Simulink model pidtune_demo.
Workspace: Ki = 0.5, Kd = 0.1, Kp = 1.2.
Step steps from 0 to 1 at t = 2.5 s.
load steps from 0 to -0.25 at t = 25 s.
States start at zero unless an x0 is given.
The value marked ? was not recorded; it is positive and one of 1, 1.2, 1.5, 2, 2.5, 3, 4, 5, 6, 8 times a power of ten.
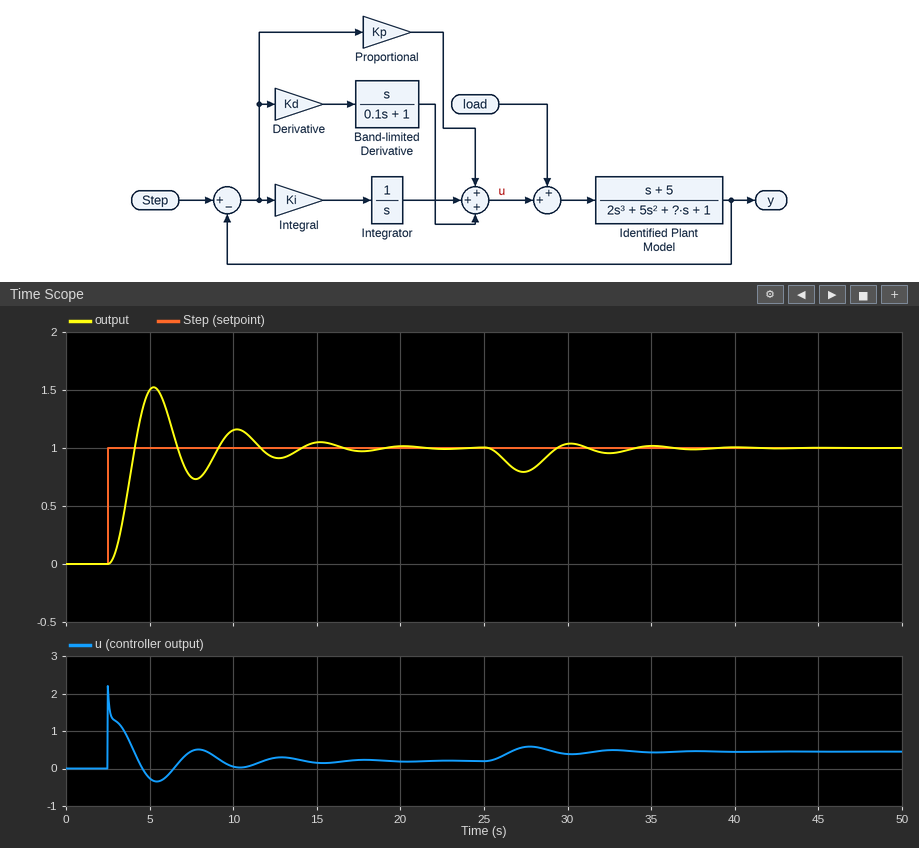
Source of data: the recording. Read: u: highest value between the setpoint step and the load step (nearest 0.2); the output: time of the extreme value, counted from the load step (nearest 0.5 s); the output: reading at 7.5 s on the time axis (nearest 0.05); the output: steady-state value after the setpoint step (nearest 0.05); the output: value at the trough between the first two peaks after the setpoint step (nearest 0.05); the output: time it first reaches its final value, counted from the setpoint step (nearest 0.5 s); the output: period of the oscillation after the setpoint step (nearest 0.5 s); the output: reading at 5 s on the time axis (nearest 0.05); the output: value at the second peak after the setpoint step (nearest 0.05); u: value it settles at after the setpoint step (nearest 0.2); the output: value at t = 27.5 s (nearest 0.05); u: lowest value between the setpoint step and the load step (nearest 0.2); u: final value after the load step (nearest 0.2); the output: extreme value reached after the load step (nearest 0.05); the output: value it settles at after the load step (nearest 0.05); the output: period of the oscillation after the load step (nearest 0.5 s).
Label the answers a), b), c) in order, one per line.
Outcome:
a) 2.2
b) 2.5 s
c) 0.75
d) 1.00
e) 0.75
f) 1.5 s
g) 5.0 s
h) 1.50
i) 1.15
j) 0.2
k) 0.80
l) -0.4
m) 0.4
n) 0.80
o) 1.00
p) 5.0 s
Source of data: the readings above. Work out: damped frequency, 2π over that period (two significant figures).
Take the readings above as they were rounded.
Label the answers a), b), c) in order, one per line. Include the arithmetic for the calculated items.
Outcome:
a) 2π / 5 = 1.3 rad/s
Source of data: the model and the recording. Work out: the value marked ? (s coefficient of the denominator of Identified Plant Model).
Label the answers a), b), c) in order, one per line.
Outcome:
a) 5
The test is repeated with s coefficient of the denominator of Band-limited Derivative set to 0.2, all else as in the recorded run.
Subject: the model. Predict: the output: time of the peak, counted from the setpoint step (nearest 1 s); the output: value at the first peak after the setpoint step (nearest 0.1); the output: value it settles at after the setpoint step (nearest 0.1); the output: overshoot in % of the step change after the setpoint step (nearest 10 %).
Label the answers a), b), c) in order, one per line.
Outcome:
a) 3 s
b) 1.5
c) 1.0
d) 50 %
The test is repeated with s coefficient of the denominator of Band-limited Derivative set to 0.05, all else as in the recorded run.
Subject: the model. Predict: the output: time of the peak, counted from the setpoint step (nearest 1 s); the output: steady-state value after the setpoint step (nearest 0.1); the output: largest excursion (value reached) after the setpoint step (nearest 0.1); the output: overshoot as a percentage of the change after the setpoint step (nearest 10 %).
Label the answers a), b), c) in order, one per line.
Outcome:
a) 3 s
b) 1.0
c) 1.5
d) 50 %
